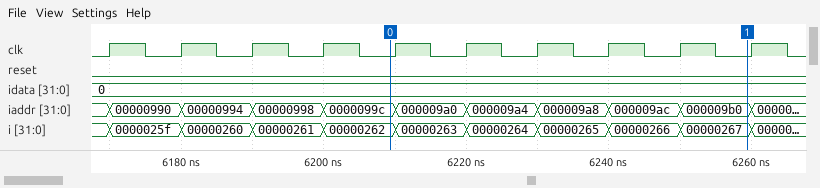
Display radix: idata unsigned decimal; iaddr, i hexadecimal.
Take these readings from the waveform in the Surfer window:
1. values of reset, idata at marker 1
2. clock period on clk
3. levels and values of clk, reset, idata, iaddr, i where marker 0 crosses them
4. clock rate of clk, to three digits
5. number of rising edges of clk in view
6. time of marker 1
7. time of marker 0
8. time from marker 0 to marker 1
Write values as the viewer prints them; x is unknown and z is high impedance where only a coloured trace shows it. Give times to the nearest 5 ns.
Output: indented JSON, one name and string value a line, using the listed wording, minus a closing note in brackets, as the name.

{
  "values of reset, idata at marker 1": "reset=0, idata=0",
  "clock period on clk": "10 ns",
  "levels and values of clk, reset, idata, iaddr, i where marker 0 crosses them": "clk=0, reset=0, idata=0, iaddr=0000099c, i=00000262",
  "clock rate of clk, to three digits": "100 MHz",
  "number of rising edges of clk in view": "10",
  "time of marker 1": "6260 ns",
  "time of marker 0": "6210 ns",
  "time from marker 0 to marker 1": "50 ns"
}
